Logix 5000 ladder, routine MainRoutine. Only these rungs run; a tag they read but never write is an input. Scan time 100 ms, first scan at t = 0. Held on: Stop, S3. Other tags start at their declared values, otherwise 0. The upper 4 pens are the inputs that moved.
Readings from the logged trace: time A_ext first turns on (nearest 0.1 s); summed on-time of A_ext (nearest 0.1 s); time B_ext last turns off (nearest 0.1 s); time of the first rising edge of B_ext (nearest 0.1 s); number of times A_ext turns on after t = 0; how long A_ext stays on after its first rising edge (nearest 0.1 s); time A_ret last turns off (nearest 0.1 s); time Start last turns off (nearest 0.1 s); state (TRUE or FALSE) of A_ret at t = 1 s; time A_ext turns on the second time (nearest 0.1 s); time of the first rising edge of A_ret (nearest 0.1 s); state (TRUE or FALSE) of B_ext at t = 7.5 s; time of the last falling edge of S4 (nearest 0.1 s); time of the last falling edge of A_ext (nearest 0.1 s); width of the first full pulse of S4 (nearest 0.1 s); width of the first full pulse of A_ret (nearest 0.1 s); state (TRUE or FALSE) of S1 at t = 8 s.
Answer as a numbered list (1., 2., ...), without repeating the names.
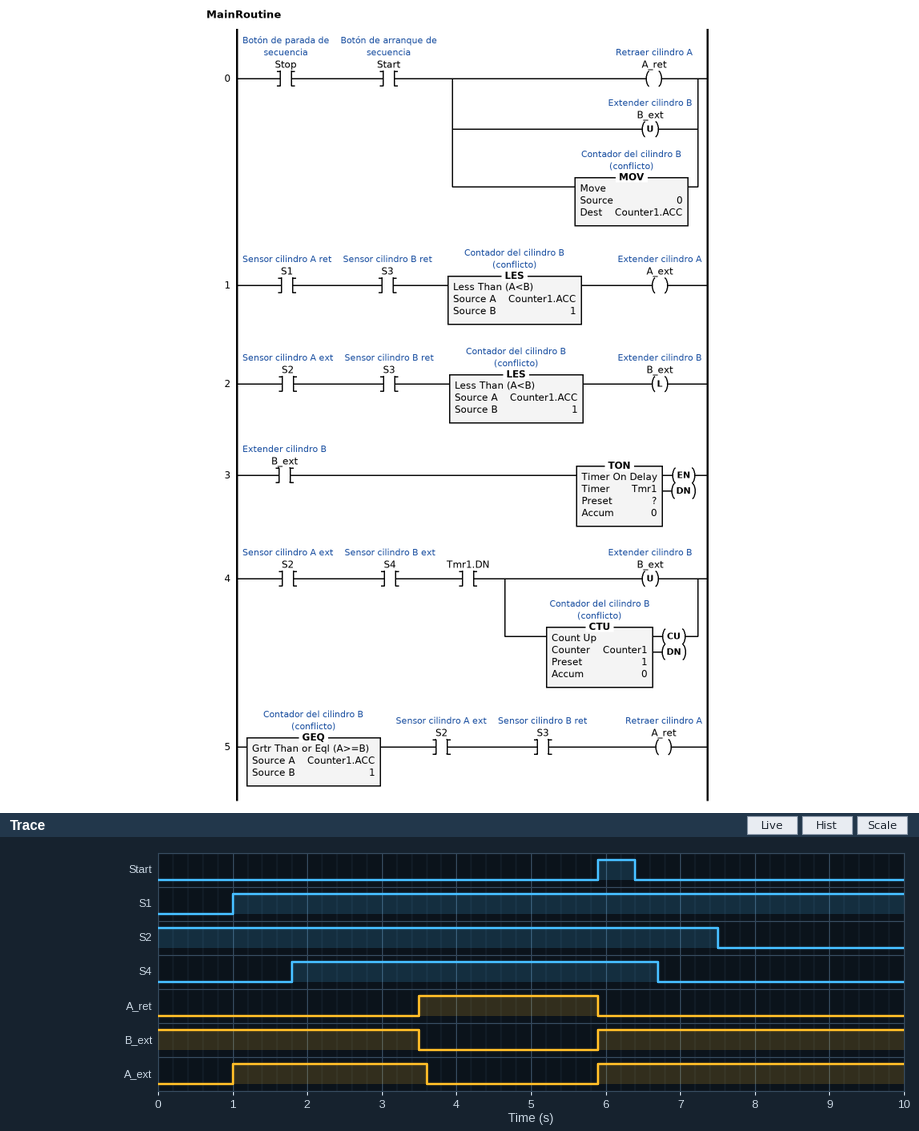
1. 1.0 s
2. 6.7 s
3. 3.5 s
4. 5.9 s
5. 2
6. 2.6 s
7. 5.9 s
8. 6.4 s
9. FALSE
10. 5.9 s
11. 3.5 s
12. TRUE
13. 6.7 s
14. 3.6 s
15. 4.9 s
16. 2.4 s
17. TRUE
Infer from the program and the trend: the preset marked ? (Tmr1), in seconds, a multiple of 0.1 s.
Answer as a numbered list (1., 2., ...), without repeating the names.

1. 3.5 s
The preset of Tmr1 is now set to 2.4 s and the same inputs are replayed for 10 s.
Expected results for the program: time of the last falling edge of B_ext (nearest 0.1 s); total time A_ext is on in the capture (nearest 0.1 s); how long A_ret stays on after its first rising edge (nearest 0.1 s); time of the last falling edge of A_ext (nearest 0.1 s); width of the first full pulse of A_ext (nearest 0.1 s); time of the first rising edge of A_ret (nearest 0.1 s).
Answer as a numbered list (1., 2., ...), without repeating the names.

1. 2.4 s
2. 5.6 s
3. 3.5 s
4. 2.5 s
5. 1.5 s
6. 2.4 s
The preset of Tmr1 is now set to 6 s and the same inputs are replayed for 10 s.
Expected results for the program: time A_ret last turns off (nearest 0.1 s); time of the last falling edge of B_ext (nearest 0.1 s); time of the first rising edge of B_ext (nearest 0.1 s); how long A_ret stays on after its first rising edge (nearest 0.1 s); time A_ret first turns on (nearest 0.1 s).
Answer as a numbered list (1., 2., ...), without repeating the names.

1. 6.1 s
2. 6.0 s
3. 6.7 s
4. 0.1 s
5. 6.0 s
